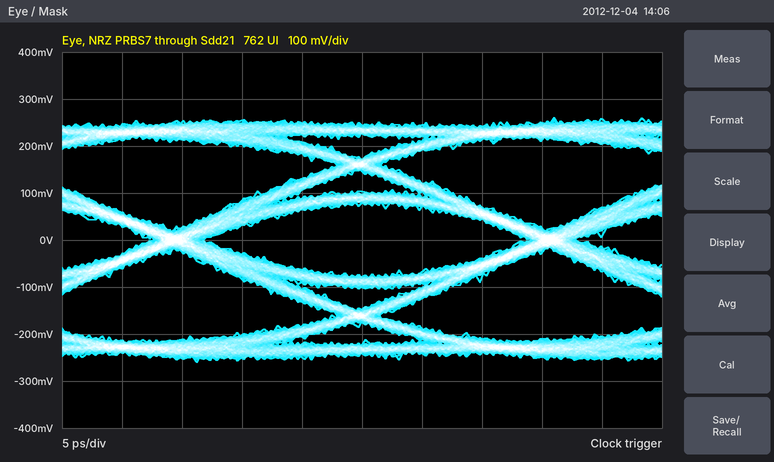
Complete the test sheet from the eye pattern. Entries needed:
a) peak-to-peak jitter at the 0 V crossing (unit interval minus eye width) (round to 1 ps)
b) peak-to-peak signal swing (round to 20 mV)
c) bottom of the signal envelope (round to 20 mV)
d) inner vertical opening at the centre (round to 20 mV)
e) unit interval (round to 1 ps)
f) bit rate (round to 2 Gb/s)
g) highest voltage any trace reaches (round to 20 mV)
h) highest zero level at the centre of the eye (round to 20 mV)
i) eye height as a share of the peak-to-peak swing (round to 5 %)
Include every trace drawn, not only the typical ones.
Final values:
4 ps
520 mV
-260 mV
160 mV
31 ps
32 Gb/s
260 mV
-80 mV
30 %
